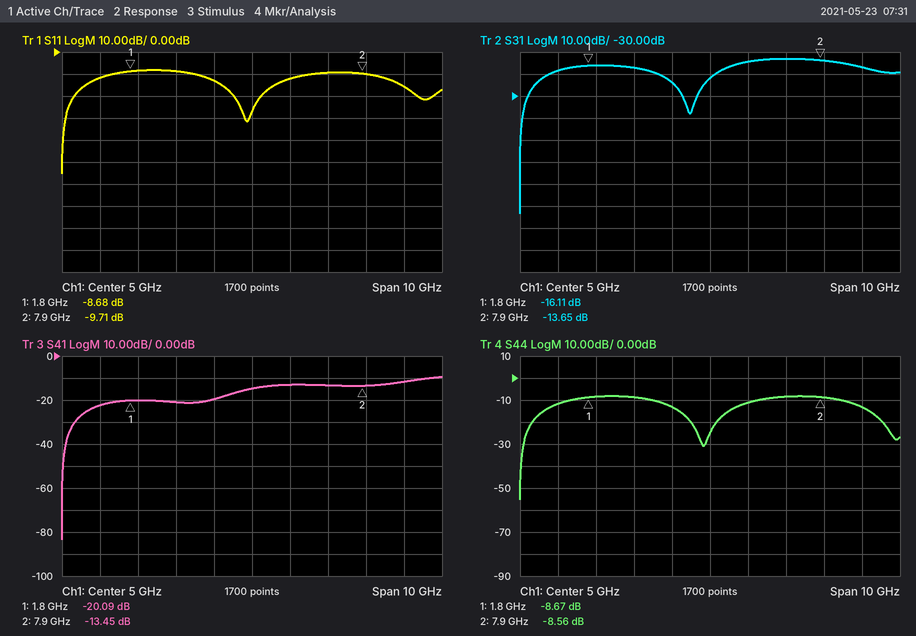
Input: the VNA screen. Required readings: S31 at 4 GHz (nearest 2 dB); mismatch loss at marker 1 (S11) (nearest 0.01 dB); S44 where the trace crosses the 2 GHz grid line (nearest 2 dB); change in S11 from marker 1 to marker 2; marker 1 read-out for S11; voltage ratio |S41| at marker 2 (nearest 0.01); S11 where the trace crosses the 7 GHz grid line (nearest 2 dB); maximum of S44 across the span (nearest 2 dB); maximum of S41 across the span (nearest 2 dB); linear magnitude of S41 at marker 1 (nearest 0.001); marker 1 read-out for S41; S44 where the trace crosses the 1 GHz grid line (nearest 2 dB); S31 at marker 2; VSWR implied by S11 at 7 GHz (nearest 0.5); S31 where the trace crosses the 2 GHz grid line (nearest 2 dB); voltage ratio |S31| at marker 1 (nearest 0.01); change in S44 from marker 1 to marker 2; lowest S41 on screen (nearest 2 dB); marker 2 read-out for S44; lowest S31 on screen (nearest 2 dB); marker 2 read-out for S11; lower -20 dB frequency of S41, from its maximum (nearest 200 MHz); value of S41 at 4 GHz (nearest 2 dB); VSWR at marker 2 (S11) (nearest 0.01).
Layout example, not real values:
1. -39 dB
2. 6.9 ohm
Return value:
1. -24 dB
2. 0.63 dB
3. -8 dB
4. -1.03 dB
5. -8.68 dB
6. 0.21
7. -10 dB
8. -8 dB
9. -10 dB
10. 0.099
11. -20.09 dB
12. -12 dB
13. -13.65 dB
14. 2.0
15. -16 dB
16. 0.16
17. 0.11 dB
18. -84 dB
19. -8.56 dB
20. -84 dB
21. -9.71 dB
22. 400 MHz
23. -20 dB
24. 1.97
